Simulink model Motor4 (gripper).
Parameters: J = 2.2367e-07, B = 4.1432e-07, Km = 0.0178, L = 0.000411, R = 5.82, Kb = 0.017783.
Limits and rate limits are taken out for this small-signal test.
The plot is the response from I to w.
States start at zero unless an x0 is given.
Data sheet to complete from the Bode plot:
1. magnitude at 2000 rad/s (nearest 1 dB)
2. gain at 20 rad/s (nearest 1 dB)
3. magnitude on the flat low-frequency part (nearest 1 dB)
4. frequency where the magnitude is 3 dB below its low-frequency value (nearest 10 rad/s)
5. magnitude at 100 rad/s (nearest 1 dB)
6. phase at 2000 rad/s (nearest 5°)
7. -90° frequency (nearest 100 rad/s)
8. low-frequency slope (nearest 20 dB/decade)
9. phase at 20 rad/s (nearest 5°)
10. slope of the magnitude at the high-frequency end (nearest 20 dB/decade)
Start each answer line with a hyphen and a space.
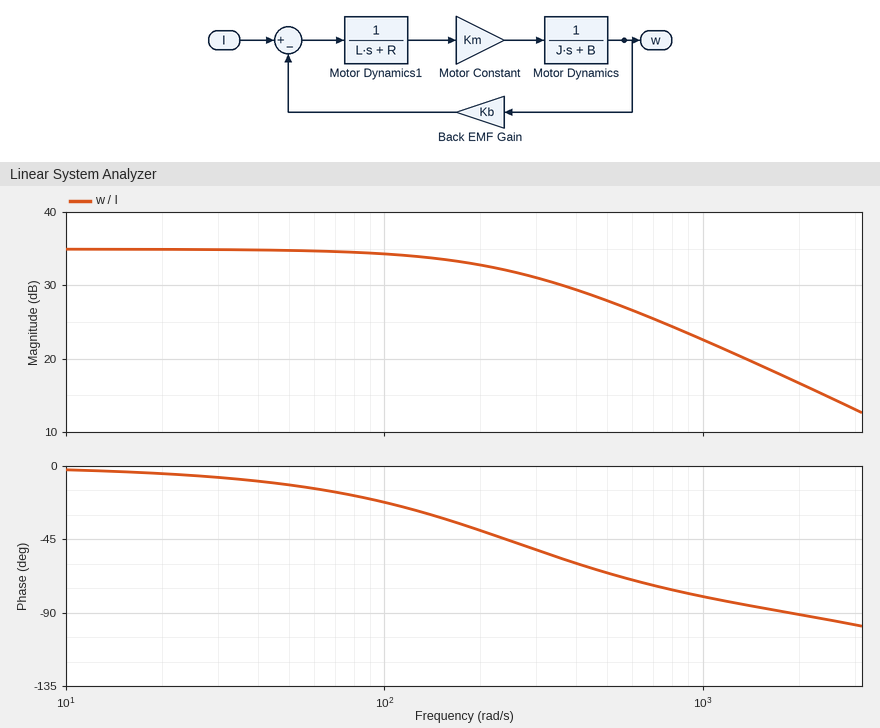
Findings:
- 17 dB
- 35 dB
- 35 dB
- 250 rad/s
- 34 dB
- -90°
- 1900 rad/s
- 0 dB/decade
- -5°
- -20 dB/decade
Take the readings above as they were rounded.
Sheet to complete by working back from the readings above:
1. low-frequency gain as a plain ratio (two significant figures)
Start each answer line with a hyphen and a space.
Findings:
- 56
